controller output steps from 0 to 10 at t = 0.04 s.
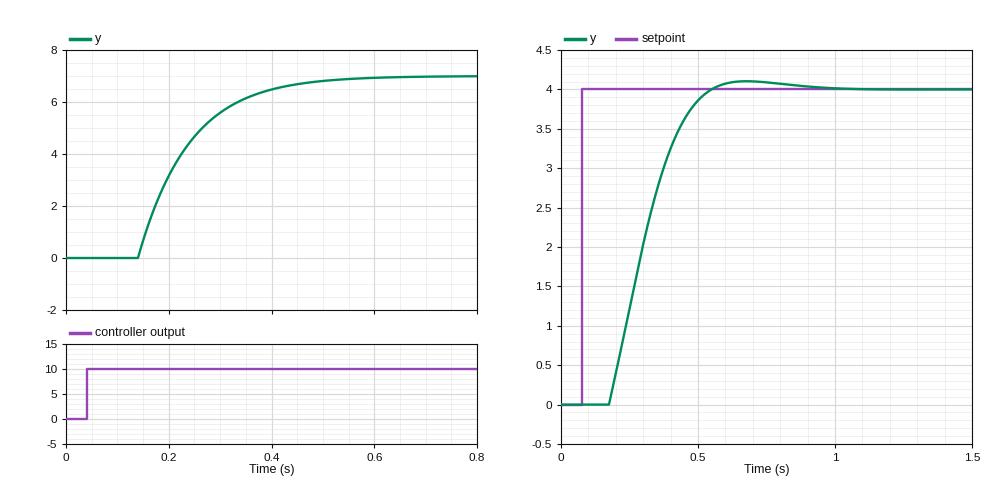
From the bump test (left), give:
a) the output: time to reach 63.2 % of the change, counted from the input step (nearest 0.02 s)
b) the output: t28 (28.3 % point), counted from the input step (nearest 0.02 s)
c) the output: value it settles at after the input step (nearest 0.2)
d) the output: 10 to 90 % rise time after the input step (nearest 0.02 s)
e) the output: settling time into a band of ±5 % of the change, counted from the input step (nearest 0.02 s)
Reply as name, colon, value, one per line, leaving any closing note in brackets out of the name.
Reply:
the output: time to reach 63.2 % of the change, counted from the input step: 0.20 s
the output: t28 (28.3 % point), counted from the input step: 0.14 s
the output: value it settles at after the input step: 7.0
the output: 10 to 90 % rise time after the input step: 0.22 s
the output: settling time into a band of ±5 % of the change, counted from the input step: 0.40 s
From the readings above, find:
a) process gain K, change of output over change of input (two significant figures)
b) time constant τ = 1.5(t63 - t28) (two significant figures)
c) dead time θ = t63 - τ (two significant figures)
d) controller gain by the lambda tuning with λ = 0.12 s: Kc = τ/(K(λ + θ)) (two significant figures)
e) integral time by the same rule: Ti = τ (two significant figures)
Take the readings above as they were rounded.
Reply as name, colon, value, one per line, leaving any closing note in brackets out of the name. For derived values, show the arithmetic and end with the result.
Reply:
process gain K, change of output over change of input: (7 - 0) / 10 = 0.70
time constant τ = 1.5(t63 - t28): 1.5 × (0.2 - 0.14) = 0.090 s
dead time θ = t63 - τ: 0.2 - 0.09 = 0.11 s
controller gain by the lambda tuning with λ = 0.12 s: Kc = τ/(K(λ + θ)): 0.09 / (0.7 × (0.12 + 0.11)) = 0.56
integral time by the same rule: Ti = τ: 0.090 s
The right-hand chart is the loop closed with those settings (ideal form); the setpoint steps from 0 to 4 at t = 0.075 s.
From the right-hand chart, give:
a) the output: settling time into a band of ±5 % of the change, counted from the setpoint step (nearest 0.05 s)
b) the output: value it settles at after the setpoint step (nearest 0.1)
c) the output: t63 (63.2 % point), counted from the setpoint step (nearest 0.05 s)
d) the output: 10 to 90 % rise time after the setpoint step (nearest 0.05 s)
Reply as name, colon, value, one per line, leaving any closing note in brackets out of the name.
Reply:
the output: settling time into a band of ±5 % of the change, counted from the setpoint step: 0.40 s
the output: value it settles at after the setpoint step: 4.0
the output: t63 (63.2 % point), counted from the setpoint step: 0.25 s
the output: 10 to 90 % rise time after the setpoint step: 0.25 s
